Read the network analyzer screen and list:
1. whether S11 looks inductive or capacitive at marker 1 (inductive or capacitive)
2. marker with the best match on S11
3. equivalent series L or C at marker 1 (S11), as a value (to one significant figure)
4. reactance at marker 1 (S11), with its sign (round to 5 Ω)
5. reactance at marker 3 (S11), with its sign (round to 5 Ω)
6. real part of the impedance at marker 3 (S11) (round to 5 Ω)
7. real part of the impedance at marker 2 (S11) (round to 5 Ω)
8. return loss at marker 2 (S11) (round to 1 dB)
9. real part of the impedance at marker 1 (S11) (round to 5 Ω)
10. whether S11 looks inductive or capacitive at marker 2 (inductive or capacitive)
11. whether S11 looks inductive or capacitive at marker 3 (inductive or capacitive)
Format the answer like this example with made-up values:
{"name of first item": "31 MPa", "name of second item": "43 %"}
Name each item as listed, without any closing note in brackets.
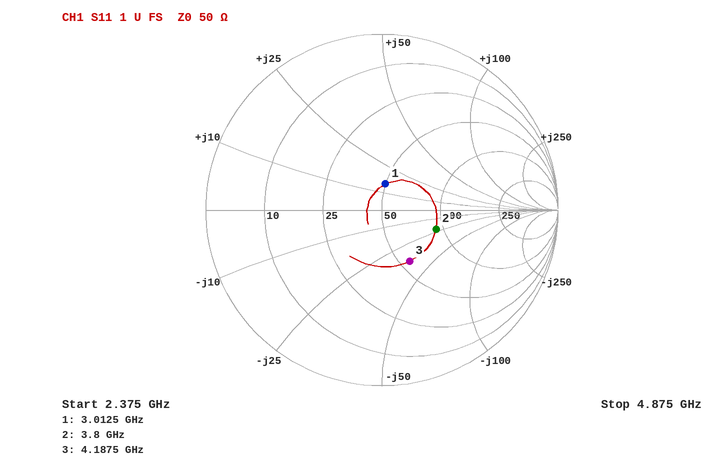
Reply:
{"whether S11 looks inductive or capacitive at marker 1": "inductive", "marker with the best match on S11": "marker 1", "equivalent series L or C at marker 1 (S11), as a value": "800 pH", "reactance at marker 1 (S11), with its sign": "+15 Ω", "reactance at marker 3 (S11), with its sign": "-35 Ω", "real part of the impedance at marker 3 (S11)": "55 Ω", "real part of the impedance at marker 2 (S11)": "90 Ω", "return loss at marker 2 (S11)": "10 dB", "real part of the impedance at marker 1 (S11)": "50 Ω", "whether S11 looks inductive or capacitive at marker 2": "capacitive", "whether S11 looks inductive or capacitive at marker 3": "capacitive"}
